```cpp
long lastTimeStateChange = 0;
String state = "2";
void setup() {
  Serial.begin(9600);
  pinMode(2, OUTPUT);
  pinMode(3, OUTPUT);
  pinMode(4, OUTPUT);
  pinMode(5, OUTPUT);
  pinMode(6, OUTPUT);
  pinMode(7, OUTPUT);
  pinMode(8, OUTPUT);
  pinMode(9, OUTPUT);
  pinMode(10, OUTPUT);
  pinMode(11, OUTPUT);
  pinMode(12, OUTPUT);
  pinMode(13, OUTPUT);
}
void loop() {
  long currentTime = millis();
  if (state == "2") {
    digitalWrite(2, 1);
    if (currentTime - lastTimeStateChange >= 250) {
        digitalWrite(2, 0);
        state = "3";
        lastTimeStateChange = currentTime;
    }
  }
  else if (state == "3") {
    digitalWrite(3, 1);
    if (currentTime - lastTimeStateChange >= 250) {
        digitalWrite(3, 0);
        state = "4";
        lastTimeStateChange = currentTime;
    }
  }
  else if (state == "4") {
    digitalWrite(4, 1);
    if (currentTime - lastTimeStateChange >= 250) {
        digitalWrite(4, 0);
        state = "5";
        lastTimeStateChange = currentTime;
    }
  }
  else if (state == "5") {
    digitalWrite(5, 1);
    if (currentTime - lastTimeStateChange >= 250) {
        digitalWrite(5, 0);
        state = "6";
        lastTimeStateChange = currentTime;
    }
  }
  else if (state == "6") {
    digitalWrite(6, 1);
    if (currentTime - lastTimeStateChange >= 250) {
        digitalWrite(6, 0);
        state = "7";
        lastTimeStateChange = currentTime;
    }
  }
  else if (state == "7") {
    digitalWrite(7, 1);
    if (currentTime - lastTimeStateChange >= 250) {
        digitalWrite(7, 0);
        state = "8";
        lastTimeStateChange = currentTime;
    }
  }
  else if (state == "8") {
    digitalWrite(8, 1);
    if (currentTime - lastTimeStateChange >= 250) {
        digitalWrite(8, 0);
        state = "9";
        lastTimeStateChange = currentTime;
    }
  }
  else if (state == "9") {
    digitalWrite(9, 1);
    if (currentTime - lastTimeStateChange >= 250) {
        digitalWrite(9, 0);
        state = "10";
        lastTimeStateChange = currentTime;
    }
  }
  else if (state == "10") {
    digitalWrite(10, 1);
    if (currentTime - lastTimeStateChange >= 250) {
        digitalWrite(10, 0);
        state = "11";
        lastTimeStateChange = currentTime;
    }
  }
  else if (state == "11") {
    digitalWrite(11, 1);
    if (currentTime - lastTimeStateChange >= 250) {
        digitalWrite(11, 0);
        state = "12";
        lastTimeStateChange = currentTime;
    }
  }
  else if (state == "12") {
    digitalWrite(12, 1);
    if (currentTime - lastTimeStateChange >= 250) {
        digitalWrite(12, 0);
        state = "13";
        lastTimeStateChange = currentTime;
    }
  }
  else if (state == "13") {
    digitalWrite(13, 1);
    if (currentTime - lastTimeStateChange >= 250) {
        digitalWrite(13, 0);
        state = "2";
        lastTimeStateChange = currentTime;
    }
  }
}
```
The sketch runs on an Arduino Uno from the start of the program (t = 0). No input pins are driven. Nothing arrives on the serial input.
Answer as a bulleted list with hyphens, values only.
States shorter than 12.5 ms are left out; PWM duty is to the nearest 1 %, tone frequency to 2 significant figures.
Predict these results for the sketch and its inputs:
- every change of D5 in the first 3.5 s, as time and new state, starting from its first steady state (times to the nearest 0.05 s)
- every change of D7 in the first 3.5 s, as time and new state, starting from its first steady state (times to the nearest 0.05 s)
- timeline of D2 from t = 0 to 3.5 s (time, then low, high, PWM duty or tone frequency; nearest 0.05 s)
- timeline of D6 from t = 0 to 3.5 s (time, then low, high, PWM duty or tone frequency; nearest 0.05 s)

- 0 s low; 0.75 s high; 1 s low
- 0 s low; 1.25 s high; 1.5 s low
- 0 s high; 0.25 s low; 3 s high; 3.25 s low
- 0 s low; 1 s high; 1.25 s low
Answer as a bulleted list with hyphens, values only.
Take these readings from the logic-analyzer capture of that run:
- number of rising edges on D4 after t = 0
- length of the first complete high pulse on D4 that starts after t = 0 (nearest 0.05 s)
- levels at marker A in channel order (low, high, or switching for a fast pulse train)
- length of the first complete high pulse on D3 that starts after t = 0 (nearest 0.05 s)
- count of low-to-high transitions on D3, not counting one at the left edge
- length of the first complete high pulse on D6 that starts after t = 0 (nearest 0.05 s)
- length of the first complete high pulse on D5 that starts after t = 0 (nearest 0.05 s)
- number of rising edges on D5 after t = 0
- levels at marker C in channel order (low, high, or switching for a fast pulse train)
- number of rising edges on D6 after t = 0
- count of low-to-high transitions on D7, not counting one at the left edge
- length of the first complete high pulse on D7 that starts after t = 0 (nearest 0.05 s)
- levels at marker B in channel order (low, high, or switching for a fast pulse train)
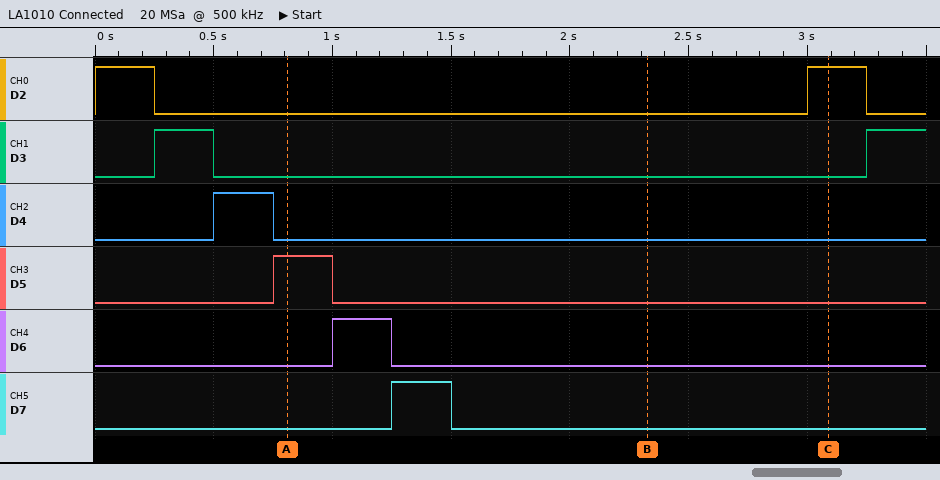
- 1
- 0.25 s
- D2 low, D3 low, D4 low, D5 high, D6 low, D7 low
- 0.25 s
- 2
- 0.25 s
- 0.25 s
- 1
- D2 high, D3 low, D4 low, D5 low, D6 low, D7 low
- 1
- 1
- 0.25 s
- D2 low, D3 low, D4 low, D5 low, D6 low, D7 low
